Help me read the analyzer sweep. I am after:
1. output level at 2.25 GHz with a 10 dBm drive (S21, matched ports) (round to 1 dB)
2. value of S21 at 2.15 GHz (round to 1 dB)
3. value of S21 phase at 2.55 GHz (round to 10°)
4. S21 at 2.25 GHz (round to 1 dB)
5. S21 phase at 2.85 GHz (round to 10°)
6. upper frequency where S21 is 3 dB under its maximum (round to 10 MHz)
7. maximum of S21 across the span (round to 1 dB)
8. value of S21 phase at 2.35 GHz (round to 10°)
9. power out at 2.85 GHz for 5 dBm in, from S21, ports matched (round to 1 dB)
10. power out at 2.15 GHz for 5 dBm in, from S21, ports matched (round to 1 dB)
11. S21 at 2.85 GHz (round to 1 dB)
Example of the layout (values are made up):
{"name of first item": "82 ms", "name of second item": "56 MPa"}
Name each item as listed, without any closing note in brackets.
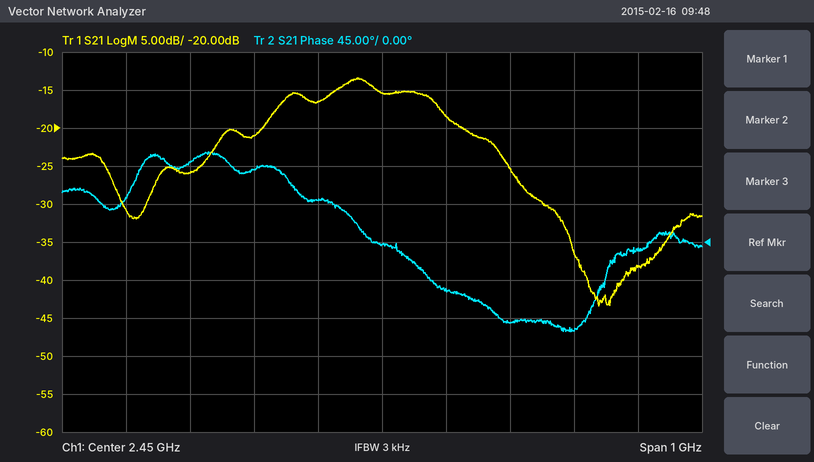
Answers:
{"output level at 2.25 GHz with a 10 dBm drive (S21, matched ports)": "-11 dBm", "value of S21 at 2.15 GHz": "-26 dB", "value of S21 phase at 2.55 GHz": "-60°", "S21 at 2.25 GHz": "-21 dB", "S21 phase at 2.85 GHz": "-10°", "upper frequency where S21 is 3 dB under its maximum": "2.53 GHz", "maximum of S21 across the span": "-13 dB", "value of S21 phase at 2.35 GHz": "50°", "power out at 2.85 GHz for 5 dBm in, from S21, ports matched": "-33 dBm", "power out at 2.15 GHz for 5 dBm in, from S21, ports matched": "-21 dBm", "S21 at 2.85 GHz": "-38 dB"}
